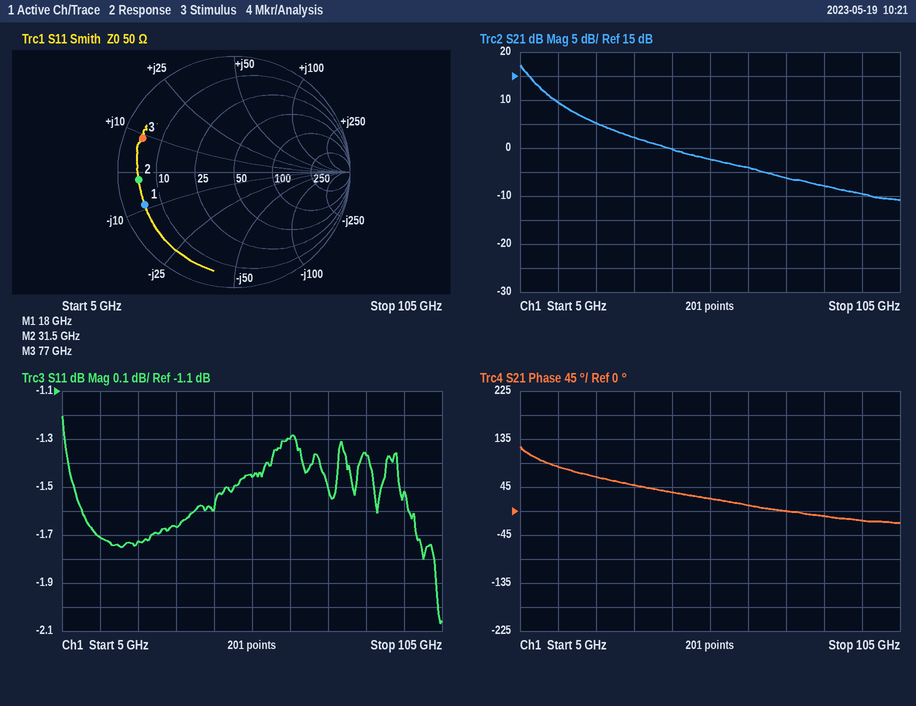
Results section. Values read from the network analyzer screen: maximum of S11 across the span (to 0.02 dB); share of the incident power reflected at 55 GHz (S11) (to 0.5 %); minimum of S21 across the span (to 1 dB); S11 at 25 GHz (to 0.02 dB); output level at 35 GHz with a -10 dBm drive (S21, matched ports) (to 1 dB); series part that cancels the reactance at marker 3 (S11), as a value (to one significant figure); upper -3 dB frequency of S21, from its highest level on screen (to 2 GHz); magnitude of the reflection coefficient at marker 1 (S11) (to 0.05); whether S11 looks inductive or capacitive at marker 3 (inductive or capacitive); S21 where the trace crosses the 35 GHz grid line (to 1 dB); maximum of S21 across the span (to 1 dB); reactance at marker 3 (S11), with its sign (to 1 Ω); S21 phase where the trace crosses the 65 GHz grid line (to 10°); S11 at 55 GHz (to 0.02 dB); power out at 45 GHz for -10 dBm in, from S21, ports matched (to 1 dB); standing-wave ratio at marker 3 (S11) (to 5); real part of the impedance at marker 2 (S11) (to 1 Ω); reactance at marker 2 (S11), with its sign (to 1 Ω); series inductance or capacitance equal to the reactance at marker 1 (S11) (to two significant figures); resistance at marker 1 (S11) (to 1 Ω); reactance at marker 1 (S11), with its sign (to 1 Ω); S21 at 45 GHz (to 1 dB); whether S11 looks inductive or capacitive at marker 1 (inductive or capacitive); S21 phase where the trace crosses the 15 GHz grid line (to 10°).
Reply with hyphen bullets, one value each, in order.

- -1.20 dB
- 71.5 %
- -11 dB
- -1.72 dB
- -8 dBm
- 200 fF
- 8 GHz
- 0.80
- inductive
- 2 dB
- 17 dB
- +9 Ω
- 10°
- -1.46 dB
- -10 dBm
- 10
- 5 Ω
- -2 Ω
- 1.0 pF
- 5 Ω
- -9 Ω
- 0 dB
- capacitive
- 80°
